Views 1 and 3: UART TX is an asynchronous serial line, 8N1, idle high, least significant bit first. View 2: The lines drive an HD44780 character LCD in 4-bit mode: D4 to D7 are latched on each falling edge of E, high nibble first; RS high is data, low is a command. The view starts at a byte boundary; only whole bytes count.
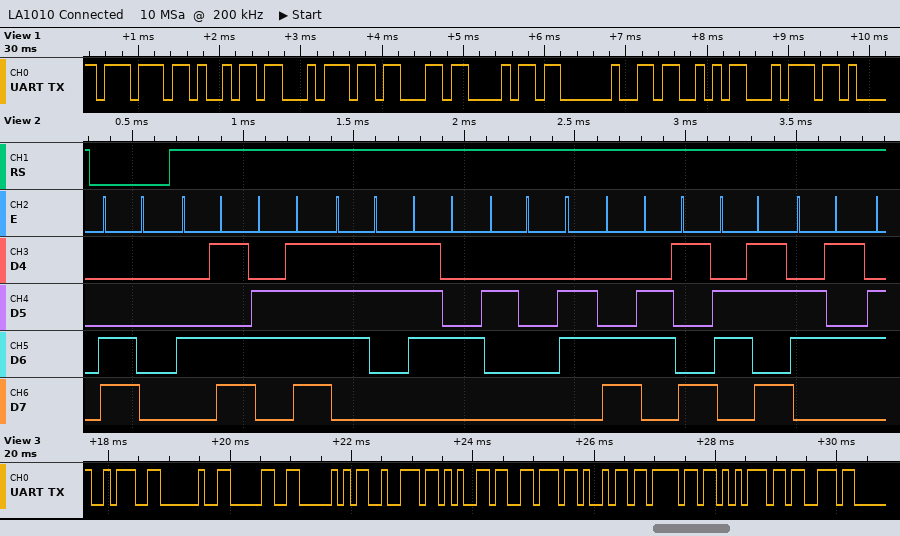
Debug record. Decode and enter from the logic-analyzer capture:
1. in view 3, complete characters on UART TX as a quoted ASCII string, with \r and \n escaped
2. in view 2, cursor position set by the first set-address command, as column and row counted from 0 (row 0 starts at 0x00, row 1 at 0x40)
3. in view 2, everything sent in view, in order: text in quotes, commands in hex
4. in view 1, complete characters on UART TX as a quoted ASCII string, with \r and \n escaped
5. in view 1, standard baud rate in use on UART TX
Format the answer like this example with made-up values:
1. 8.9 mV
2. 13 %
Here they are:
1. ": 0Previous"
2. column 0, row 1
3. 0xC0 "Most like"
4. "witch St"
5. 9600 baud
